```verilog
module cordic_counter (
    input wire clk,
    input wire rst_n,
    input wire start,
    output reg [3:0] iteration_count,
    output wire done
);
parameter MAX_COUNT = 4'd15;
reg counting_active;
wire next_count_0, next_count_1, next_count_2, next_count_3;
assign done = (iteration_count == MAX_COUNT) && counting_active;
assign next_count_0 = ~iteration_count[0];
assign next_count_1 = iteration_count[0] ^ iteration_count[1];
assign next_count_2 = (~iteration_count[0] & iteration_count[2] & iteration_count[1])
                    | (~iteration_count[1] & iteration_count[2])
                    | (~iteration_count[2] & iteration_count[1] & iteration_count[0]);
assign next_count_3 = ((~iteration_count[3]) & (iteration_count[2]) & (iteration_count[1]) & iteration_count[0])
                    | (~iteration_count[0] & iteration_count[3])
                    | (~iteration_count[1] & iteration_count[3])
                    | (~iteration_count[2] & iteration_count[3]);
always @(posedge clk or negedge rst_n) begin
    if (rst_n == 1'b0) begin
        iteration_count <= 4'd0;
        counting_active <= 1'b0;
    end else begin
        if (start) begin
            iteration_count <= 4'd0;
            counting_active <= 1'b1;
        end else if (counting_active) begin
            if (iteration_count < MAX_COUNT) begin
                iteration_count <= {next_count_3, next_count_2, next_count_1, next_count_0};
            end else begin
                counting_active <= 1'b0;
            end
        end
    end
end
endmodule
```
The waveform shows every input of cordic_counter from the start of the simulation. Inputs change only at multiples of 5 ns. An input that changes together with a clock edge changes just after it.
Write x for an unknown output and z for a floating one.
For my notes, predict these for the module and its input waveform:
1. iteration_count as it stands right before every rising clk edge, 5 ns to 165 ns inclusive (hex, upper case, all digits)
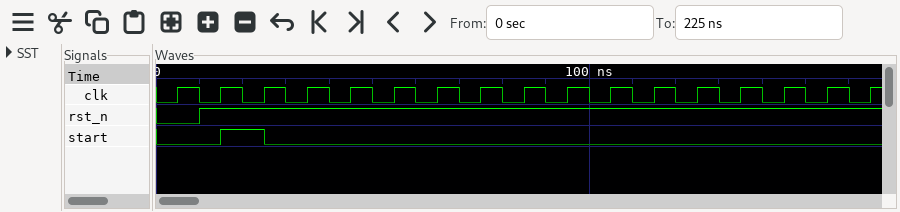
0, 0, 0, 0, 1, 2, 3, 4, 5, 6, 7, 8, 9, A, B, C, D
